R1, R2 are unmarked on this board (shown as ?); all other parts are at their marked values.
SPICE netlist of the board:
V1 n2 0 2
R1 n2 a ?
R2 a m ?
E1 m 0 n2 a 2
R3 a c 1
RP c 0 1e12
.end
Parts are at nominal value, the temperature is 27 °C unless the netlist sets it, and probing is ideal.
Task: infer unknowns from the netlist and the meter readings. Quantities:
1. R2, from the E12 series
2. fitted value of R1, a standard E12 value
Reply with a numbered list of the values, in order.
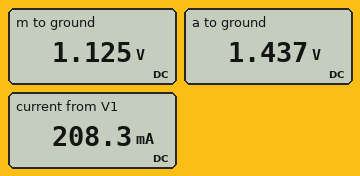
1. 1.5 Ω
2. 2.7 Ω
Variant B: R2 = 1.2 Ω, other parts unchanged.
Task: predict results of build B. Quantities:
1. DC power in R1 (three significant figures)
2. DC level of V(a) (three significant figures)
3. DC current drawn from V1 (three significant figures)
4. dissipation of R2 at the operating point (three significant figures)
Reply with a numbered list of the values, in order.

1. 125 mW
2. 1.42 V
3. 215 mA
4. 55.5 mW
